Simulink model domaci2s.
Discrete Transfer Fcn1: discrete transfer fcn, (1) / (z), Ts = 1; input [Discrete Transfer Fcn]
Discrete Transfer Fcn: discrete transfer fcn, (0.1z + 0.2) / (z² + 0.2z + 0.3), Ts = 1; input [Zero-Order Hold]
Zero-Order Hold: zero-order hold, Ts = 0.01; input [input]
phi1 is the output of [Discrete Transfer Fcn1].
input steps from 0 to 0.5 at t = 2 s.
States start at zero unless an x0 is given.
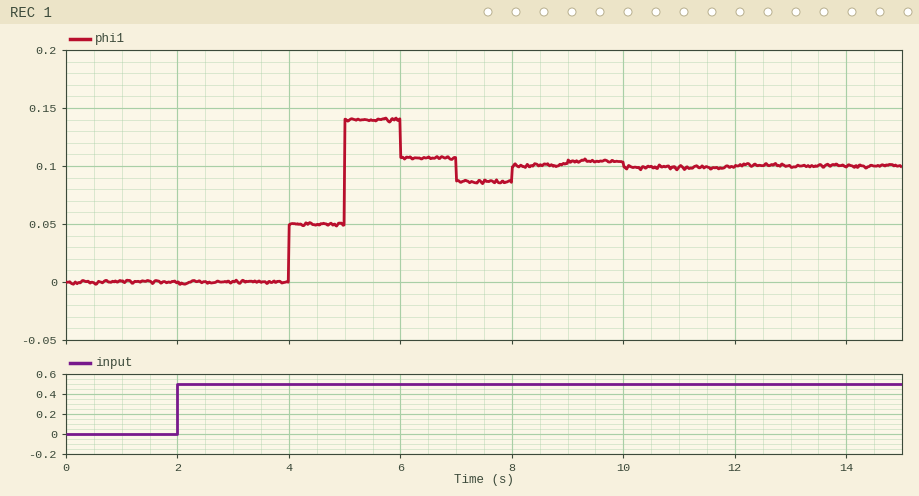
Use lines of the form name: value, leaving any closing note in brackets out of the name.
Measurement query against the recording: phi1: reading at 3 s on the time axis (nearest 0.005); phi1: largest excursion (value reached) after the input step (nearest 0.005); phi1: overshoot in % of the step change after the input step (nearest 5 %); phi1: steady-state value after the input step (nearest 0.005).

phi1: reading at 3 s on the time axis: 0.000
phi1: largest excursion (value reached) after the input step: 0.140
phi1: overshoot in % of the step change after the input step: 40 %
phi1: steady-state value after the input step: 0.100
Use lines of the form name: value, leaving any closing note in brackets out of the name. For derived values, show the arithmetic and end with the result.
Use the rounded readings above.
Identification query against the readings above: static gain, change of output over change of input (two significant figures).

static gain, change of output over change of input: (0.1 - 0) / (0.5 - 0) = 0.20
